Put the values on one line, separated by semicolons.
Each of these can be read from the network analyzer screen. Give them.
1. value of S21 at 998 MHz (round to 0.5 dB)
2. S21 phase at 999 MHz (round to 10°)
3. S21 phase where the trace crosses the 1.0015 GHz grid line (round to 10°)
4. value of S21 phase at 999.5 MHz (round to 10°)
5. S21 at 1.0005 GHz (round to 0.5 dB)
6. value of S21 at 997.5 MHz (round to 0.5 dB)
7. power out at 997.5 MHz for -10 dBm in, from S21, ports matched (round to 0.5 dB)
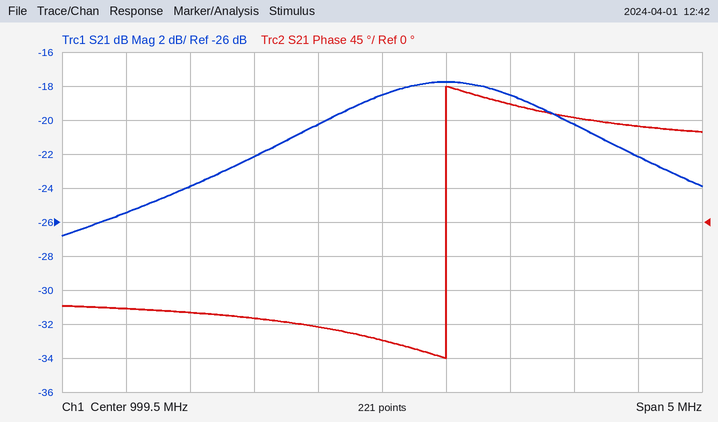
-24.0 dB; -140°; 130°; -160°; -18.5 dB; -25.5 dB; -35.5 dBm
